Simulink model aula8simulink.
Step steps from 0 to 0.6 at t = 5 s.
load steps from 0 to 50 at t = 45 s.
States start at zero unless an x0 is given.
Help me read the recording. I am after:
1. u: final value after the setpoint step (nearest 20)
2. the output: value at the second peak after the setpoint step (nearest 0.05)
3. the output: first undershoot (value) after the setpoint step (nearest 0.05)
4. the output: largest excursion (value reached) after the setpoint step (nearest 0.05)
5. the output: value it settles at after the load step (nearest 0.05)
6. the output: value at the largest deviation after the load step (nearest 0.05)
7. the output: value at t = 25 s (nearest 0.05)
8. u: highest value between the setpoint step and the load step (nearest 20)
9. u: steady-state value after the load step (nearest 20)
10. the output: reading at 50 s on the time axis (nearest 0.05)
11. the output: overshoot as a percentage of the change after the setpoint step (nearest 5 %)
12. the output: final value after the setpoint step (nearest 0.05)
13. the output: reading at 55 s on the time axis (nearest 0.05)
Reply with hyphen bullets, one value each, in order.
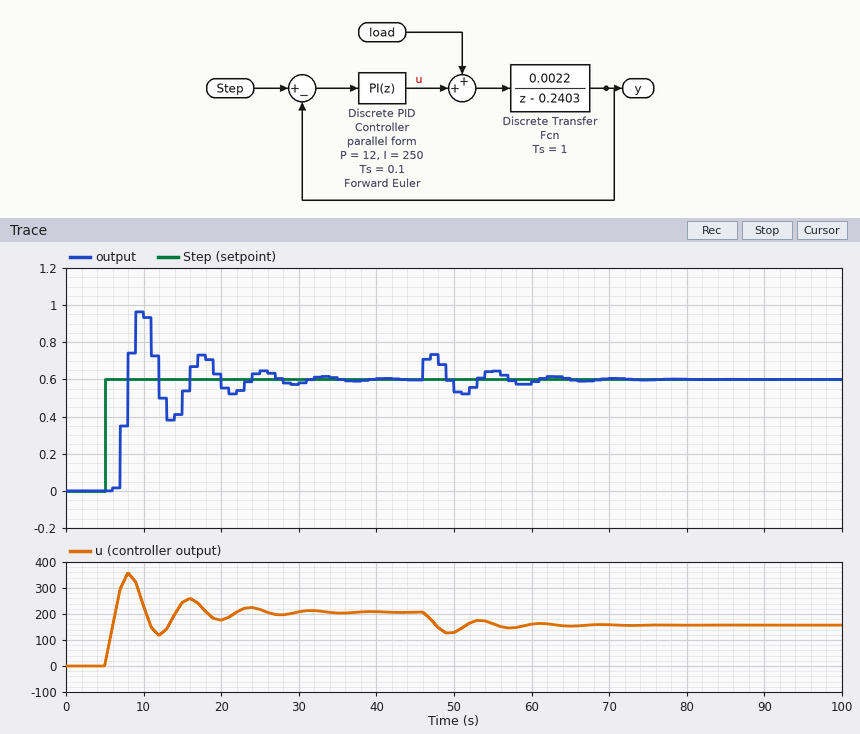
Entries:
- 200
- 0.75
- 0.40
- 0.95
- 0.60
- 0.75
- 0.65
- 360
- 160
- 0.55
- 60 %
- 0.60
- 0.65
